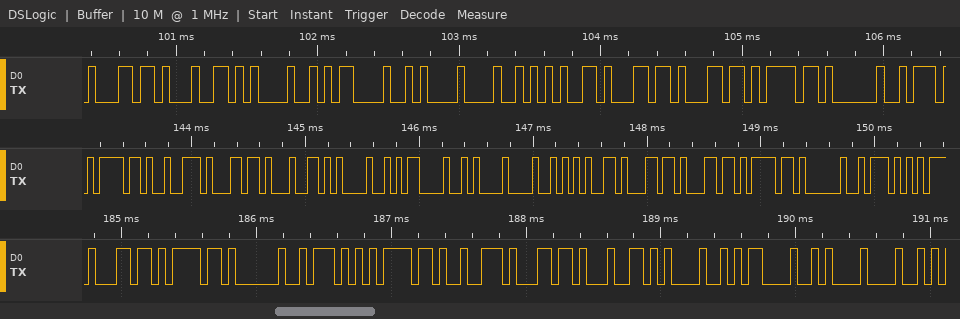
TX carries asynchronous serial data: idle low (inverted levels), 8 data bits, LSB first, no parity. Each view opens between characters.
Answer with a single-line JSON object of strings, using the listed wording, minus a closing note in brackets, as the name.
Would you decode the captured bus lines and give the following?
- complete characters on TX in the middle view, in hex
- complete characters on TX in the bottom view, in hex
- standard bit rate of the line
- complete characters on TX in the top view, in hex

{"complete characters on TX in the middle view, in hex": "21, 1B, 27, 37, BD, E5, EB, 6F, 35, 27, 27, 21, BF, 51", "complete characters on TX in the bottom view, in hex": "27, 21, BF, 51, 21, 1B, 27, 37, BD, E5, EB, 6F", "standard bit rate of the line": "19200 baud", "complete characters on TX in the top view, in hex": "27, 37, BD, E5, EB, 6F, 35, 27, 27, 21, BF"}
